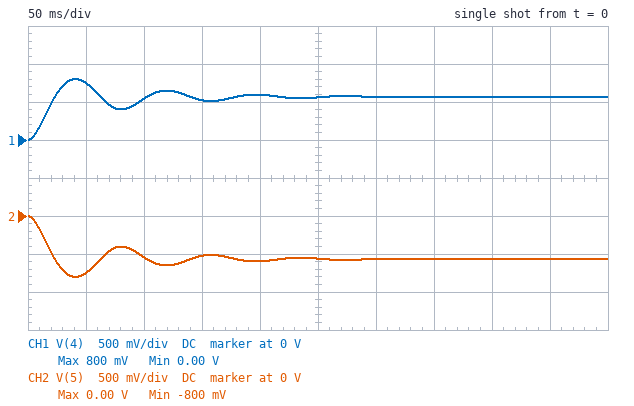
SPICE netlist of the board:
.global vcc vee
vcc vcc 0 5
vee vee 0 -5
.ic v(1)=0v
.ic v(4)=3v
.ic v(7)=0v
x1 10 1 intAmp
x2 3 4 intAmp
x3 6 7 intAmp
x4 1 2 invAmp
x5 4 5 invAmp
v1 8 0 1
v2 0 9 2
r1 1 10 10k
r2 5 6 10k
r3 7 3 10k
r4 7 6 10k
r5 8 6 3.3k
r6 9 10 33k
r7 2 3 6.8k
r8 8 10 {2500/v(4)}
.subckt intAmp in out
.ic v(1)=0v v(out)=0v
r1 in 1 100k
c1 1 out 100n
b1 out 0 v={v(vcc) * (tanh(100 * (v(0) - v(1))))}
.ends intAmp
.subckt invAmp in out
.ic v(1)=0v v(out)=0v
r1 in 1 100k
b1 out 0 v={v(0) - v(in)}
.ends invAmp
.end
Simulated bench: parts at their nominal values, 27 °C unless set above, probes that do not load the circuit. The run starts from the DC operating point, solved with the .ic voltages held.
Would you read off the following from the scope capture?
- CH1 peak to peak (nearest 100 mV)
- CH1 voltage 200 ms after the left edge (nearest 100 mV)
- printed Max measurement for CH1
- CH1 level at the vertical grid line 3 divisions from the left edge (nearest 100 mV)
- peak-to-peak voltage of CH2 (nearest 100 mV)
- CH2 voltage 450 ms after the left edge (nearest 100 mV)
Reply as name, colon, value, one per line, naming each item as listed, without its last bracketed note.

CH1 peak to peak: 800 mV
CH1 voltage 200 ms after the left edge: 600 mV
printed Max measurement for CH1: 800 mV
CH1 level at the vertical grid line 3 divisions from the left edge: 500 mV
peak-to-peak voltage of CH2: 800 mV
CH2 voltage 450 ms after the left edge: -600 mV
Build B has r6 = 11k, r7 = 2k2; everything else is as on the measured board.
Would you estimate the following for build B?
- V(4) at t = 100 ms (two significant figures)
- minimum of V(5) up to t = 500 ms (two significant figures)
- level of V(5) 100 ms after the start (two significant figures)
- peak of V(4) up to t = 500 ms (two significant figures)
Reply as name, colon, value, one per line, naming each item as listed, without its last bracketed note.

V(4) at t = 100 ms: 730 mV
minimum of V(5) up to t = 500 ms: -1.1 V
level of V(5) 100 ms after the start: -730 mV
peak of V(4) up to t = 500 ms: 1.1 V
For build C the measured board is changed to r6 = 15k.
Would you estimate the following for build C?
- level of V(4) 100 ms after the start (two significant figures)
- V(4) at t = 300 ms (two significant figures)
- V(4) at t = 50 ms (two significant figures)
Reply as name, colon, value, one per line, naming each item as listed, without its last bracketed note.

level of V(4) 100 ms after the start: 530 mV
V(4) at t = 300 ms: 750 mV
V(4) at t = 50 ms: 1.2 V
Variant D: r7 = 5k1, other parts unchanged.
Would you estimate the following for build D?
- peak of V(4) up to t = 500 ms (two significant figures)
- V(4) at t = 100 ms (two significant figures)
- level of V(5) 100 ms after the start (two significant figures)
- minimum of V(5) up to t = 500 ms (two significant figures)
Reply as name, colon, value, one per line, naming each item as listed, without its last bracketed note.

peak of V(4) up to t = 500 ms: 640 mV
V(4) at t = 100 ms: 520 mV
level of V(5) 100 ms after the start: -520 mV
minimum of V(5) up to t = 500 ms: -640 mV
